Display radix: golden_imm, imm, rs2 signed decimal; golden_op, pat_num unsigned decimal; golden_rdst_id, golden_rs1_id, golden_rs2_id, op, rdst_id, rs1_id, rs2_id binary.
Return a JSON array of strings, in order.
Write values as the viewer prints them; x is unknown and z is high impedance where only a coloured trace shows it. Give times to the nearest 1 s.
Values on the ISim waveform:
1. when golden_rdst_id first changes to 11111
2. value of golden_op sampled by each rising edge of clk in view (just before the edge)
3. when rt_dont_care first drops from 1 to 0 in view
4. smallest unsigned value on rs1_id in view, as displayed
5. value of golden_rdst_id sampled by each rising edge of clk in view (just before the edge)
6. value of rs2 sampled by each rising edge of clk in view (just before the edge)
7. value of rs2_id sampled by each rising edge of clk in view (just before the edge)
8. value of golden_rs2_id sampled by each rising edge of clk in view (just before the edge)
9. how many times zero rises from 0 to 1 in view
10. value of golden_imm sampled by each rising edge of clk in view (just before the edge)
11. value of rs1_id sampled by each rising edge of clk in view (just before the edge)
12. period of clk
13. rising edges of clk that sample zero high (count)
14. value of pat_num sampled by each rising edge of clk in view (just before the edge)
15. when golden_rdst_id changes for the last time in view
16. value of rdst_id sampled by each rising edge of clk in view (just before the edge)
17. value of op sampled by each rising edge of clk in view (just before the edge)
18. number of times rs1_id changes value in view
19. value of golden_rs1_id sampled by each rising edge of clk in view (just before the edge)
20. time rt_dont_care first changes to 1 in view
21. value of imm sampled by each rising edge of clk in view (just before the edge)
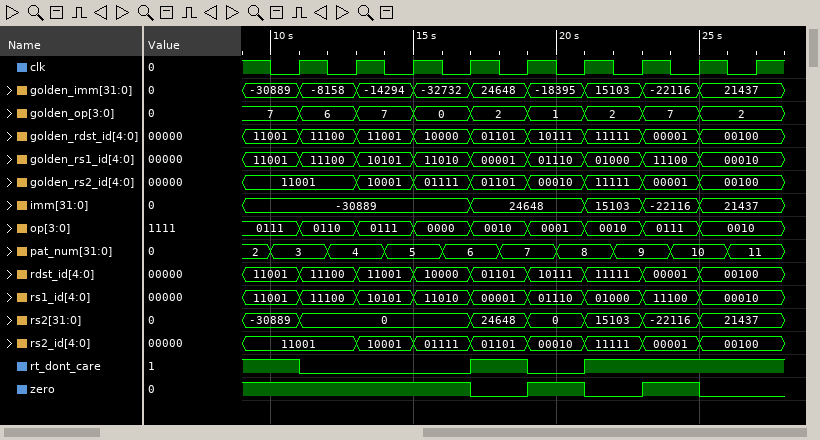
["21 s", "7, 6, 7, 0, 2, 1, 2, 7, 2", "11 s", "00001", "11001, 11100, 11001, 10000, 01101, 10111, 11111, 00001, 00100", "-30889, 0, 0, 0, 24648, 0, 15103, -22116, 21437", "11001, 11001, 10001, 01111, 01101, 00010, 11111, 00001, 00100", "11001, 11001, 10001, 01111, 01101, 00010, 11111, 00001, 00100", "2", "-30889, -8158, -14294, -32732, 24648, -18395, 15103, -22116, 21437", "11001, 11100, 10101, 11010, 00001, 01110, 01000, 11100, 00010", "2 s", "6", "3, 4, 5, 6, 7, 8, 9, 10, 11", "25 s", "11001, 11100, 11001, 10000, 01101, 10111, 11111, 00001, 00100", "0111, 0110, 0111, 0000, 0010, 0001, 0010, 0111, 0010", "8", "11001, 11100, 10101, 11010, 00001, 01110, 01000, 11100, 00010", "17 s", "-30889, -30889, -30889, -30889, 24648, 24648, 15103, -22116, 21437"]
